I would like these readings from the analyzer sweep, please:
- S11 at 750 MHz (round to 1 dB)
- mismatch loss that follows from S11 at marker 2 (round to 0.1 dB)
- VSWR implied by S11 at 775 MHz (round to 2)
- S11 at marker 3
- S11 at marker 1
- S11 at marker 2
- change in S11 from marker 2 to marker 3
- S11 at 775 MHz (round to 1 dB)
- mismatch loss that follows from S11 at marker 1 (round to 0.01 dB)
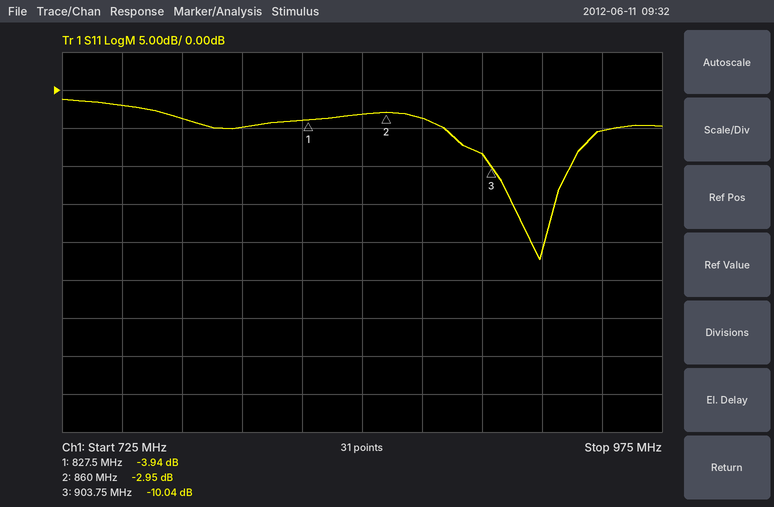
-2 dB
3.1 dB
4
-10.04 dB
-3.94 dB
-2.95 dB
-7.09 dB
-4 dB
2.24 dB
